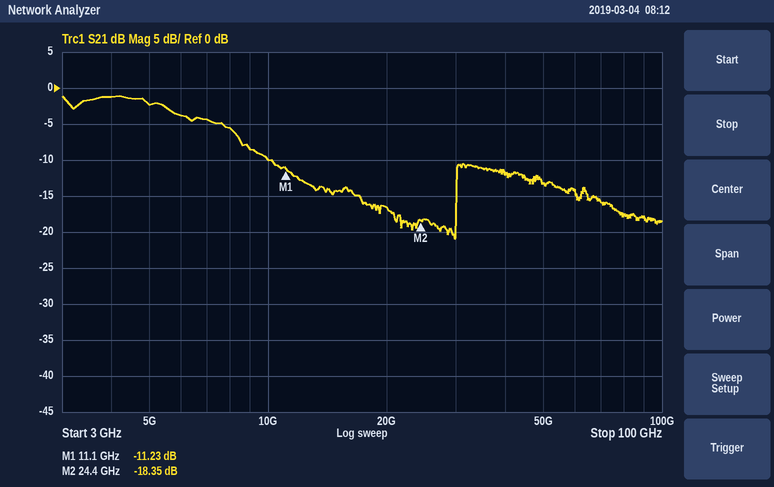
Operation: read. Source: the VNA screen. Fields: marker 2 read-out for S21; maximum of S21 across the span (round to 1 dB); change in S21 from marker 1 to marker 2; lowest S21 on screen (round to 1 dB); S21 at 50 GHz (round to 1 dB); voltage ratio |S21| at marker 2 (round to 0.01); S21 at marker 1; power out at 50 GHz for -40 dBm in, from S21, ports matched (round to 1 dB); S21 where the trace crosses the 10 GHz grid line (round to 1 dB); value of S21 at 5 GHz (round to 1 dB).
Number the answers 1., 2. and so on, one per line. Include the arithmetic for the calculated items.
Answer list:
1. -18.35 dB
2. -1 dB
3. -18.35 − (-11.23) = -7.12 dB
4. -21 dB
5. -13 dB
6. 10^(-18.35/20) ≈ 0.12
7. -11.23 dB
8. -40 dBm + (-13 dB) = -53 dBm
9. -10 dB
10. -2 dB
